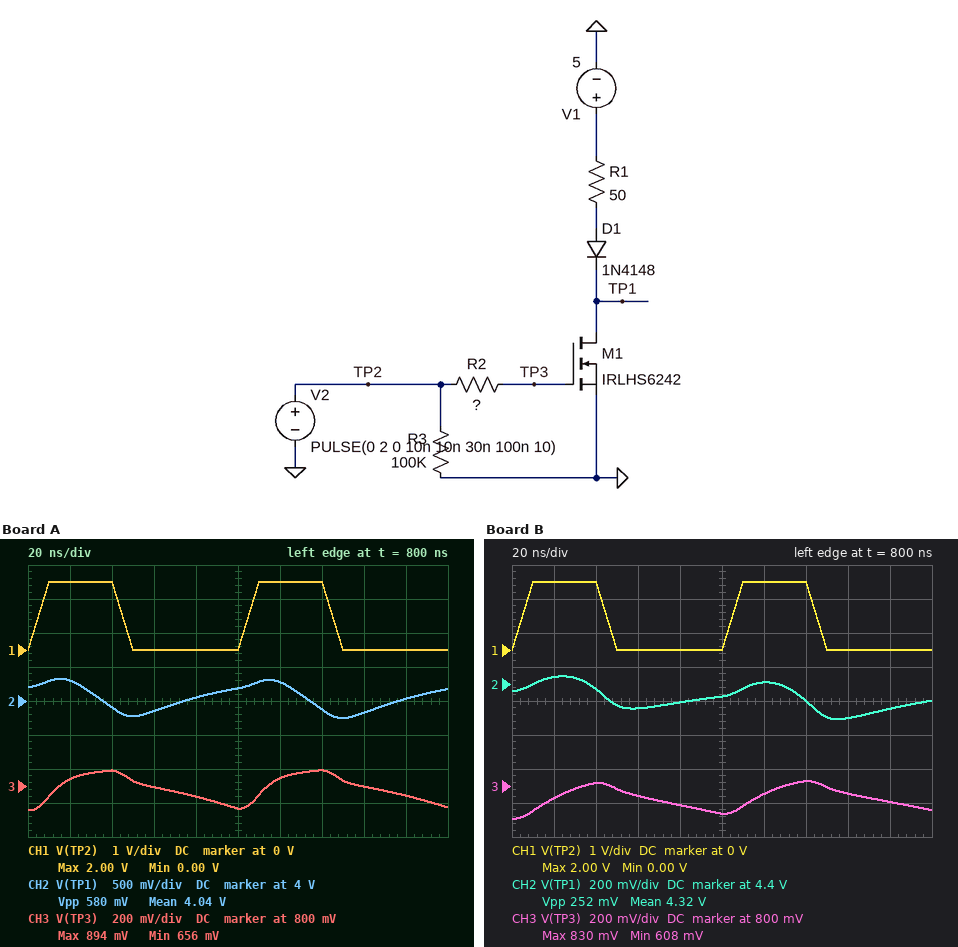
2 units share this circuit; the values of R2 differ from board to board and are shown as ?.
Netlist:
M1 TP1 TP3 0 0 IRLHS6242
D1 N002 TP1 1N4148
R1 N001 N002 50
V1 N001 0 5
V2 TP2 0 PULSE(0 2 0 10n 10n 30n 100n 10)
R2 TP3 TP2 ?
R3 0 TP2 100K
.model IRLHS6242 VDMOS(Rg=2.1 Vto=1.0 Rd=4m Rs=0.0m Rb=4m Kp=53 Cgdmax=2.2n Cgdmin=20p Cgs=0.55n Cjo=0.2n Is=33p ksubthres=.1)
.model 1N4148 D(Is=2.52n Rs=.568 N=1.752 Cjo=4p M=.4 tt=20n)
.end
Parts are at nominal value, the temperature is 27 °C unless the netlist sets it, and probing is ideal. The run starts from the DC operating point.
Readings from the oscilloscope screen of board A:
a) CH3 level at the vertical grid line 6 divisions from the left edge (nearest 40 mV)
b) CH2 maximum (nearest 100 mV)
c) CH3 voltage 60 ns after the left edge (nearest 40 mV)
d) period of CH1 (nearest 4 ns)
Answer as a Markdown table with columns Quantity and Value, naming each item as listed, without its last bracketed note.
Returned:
| Quantity | Value |
|---|---|
| CH3 level at the vertical grid line 6 divisions from the left edge | 840 mV |
| CH2 maximum | 4.3 V |
| CH3 voltage 60 ns after the left edge | 800 mV |
| period of CH1 | 100 ns |
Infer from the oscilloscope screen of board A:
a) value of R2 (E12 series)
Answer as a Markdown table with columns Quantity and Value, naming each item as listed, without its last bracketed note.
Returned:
| Quantity | Value |
|---|---|
| value of R2 | 150 Ω |
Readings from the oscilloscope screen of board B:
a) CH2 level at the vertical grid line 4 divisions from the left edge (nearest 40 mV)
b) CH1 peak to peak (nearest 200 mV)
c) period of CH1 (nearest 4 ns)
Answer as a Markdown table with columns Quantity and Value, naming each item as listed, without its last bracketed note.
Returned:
| Quantity | Value |
|---|---|
| CH2 level at the vertical grid line 4 divisions from the left edge | 4.28 V |
| CH1 peak to peak | 2.0 V |
| period of CH1 | 100 ns |
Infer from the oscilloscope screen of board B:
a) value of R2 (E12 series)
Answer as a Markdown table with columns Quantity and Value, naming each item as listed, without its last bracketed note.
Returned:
| Quantity | Value |
|---|---|
| value of R2 | 270 Ω |
